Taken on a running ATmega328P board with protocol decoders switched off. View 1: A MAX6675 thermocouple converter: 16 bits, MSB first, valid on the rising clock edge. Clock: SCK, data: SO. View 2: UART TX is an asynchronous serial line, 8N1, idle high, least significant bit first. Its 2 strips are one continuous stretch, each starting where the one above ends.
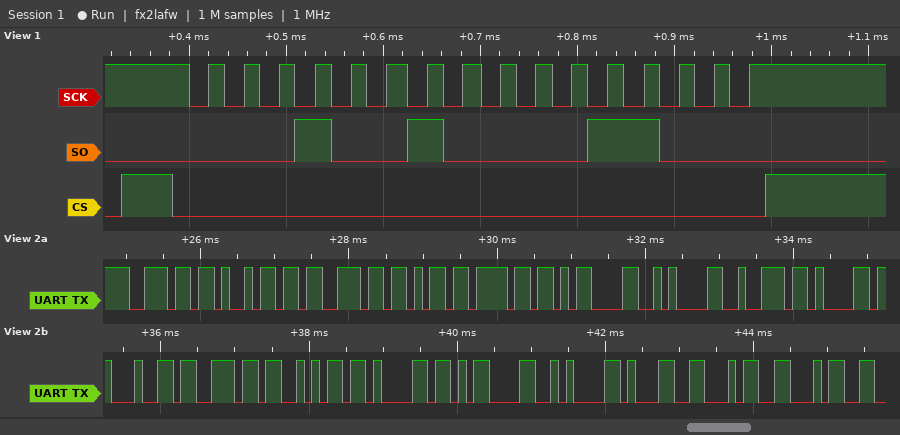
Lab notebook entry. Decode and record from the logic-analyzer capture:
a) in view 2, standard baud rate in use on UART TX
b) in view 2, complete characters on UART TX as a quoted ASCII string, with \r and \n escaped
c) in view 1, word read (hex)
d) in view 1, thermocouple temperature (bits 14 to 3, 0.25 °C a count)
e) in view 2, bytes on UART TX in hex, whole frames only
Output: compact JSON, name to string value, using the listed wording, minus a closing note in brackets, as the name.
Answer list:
{"in view 2, standard baud rate in use on UART TX": "9600 baud", "in view 2, complete characters on UART TX as a quoted ASCII string, with \\r and \\n escaped": "\"nisko\\r\\nradnja\\r\\n144\"", "in view 1, word read": "0x1218", "in view 1, thermocouple temperature": "144.75 °C", "in view 2, bytes on UART TX in hex, whole frames only": "6E 69 73 6B 6F 0D 0A 72 61 64 6E 6A 61 0D 0A 31 34 34"}
